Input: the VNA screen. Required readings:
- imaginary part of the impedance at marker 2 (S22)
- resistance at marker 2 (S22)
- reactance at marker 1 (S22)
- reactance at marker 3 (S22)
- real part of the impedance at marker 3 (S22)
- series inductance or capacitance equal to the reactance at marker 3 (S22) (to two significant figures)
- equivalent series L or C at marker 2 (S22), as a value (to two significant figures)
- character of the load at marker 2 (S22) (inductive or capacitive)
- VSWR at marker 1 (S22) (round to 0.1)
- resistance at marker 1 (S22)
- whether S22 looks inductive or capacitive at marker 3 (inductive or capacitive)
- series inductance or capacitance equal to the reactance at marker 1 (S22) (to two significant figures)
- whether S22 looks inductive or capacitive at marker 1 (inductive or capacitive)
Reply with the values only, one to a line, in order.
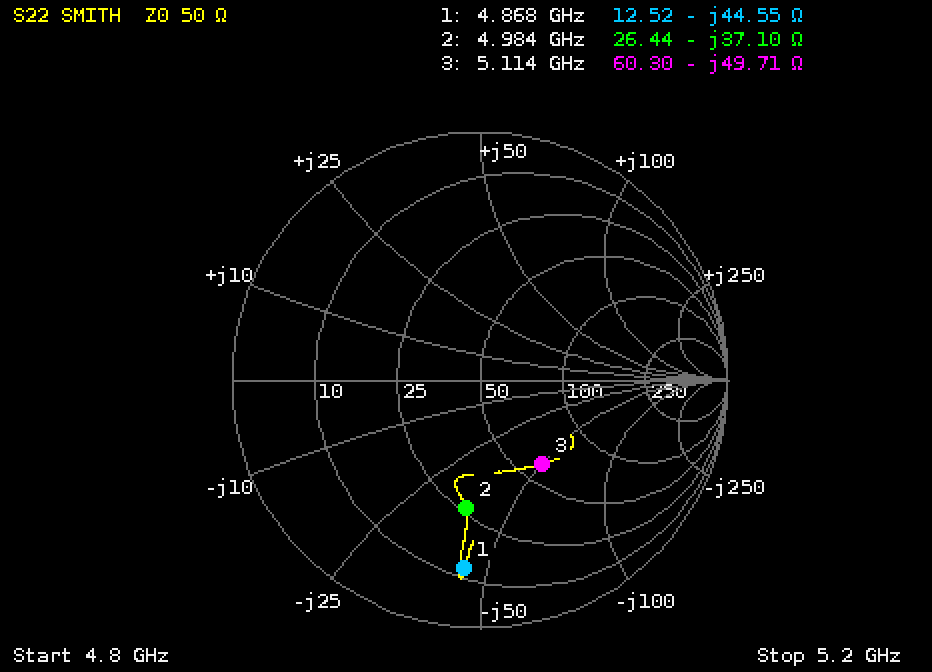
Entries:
-37.10 Ω
26.44 Ω
-44.55 Ω
-49.71 Ω
60.30 Ω
630 fF
860 fF
capacitive
7.3
12.52 Ω
capacitive
730 fF
capacitive
